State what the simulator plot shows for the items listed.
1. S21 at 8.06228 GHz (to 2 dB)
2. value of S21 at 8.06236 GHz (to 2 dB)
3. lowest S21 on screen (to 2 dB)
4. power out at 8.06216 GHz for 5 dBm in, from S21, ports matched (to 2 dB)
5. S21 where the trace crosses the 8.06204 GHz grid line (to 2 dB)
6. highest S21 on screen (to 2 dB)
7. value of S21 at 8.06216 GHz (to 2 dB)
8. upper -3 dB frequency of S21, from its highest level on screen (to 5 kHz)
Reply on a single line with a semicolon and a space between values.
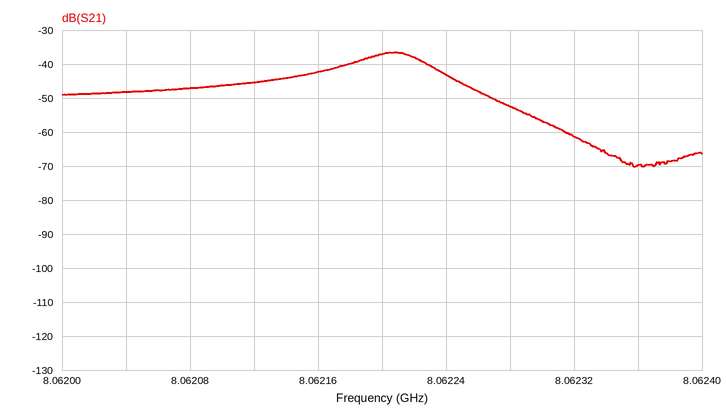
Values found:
-52 dB; -70 dB; -70 dB; -38 dBm; -48 dB; -36 dB; -42 dB; 8.062225 GHz
